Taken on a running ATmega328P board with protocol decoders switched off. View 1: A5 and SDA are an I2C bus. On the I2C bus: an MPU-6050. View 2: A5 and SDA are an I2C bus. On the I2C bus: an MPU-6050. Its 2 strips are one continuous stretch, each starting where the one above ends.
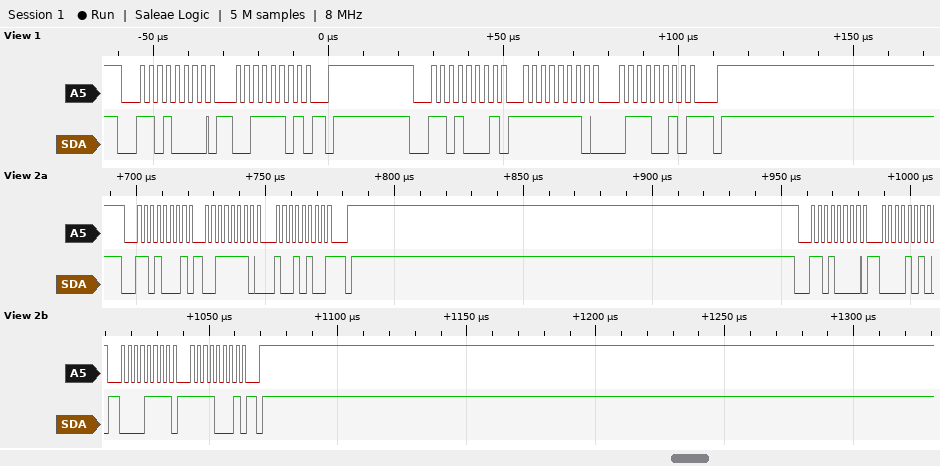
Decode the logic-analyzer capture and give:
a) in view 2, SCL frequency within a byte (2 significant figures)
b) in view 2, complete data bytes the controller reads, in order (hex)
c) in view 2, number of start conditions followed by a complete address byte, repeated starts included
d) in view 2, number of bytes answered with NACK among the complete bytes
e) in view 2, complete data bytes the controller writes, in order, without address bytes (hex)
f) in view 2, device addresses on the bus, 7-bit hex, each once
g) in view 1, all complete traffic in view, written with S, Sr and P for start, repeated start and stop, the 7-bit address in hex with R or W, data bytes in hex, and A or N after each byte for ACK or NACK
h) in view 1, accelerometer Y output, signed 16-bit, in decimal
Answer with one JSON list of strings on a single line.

["400 kHz", "3E 94", "2", "1", "0A 0F F1", "0x68", "S 68W A 3D A P S 68R A FE A 72 N P", "-398"]
